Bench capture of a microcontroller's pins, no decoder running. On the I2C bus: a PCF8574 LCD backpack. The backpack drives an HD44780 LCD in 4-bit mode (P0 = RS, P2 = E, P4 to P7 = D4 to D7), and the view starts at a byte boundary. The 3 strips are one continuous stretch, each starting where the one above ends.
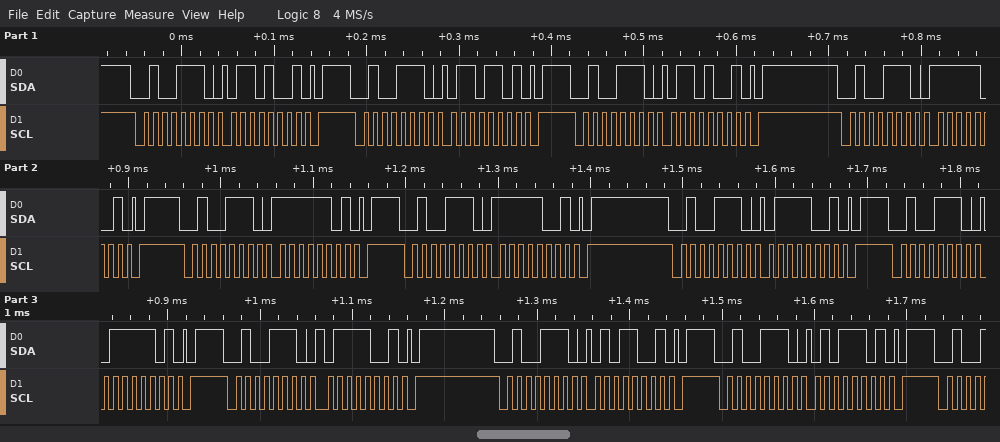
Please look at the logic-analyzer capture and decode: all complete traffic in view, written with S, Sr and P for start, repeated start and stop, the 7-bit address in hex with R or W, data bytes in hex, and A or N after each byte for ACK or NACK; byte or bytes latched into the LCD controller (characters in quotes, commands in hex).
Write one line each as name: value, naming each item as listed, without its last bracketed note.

all complete traffic in view, written with S, Sr and P for start, repeated start and stop, the 7-bit address in hex with R or W, data bytes in hex, and A or N after each byte for ACK or NACK: S 27W A 69 A P S 27W A 6D A P S 27W A 69 A P S 27W A F9 A P S 27W A FD A P S 27W A F9 A P S 27W A 79 A P S 27W A 7D A P S 27W A 79 A P S 27W A 59 A P S 27W A 5D A P
byte or bytes latched into the LCD controller: 'o'
